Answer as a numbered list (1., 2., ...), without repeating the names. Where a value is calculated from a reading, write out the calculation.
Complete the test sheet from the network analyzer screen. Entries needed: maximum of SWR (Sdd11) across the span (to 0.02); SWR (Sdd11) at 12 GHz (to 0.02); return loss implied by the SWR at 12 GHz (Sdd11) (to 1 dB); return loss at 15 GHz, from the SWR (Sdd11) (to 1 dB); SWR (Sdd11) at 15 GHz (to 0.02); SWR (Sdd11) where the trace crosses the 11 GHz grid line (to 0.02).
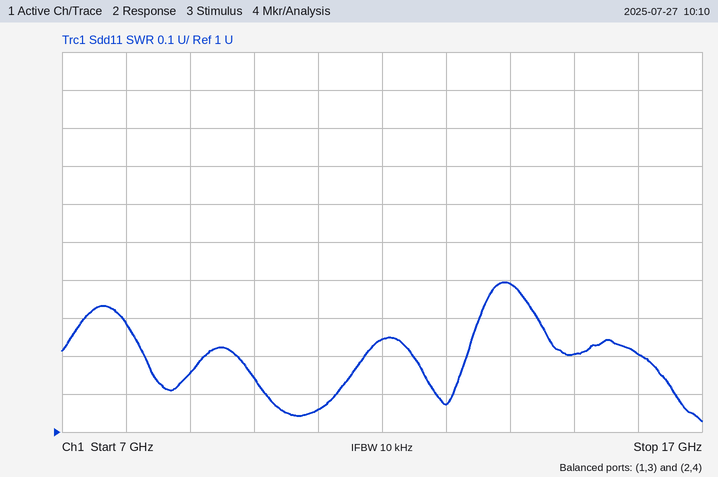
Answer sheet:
1. 1.40
2. 1.24
3. −20 log10((1.24 − 1)/(1.24 + 1)) ≈ 19 dB
4. −20 log10((1.2 − 1)/(1.2 + 1)) ≈ 21 dB
5. 1.20
6. 1.06
